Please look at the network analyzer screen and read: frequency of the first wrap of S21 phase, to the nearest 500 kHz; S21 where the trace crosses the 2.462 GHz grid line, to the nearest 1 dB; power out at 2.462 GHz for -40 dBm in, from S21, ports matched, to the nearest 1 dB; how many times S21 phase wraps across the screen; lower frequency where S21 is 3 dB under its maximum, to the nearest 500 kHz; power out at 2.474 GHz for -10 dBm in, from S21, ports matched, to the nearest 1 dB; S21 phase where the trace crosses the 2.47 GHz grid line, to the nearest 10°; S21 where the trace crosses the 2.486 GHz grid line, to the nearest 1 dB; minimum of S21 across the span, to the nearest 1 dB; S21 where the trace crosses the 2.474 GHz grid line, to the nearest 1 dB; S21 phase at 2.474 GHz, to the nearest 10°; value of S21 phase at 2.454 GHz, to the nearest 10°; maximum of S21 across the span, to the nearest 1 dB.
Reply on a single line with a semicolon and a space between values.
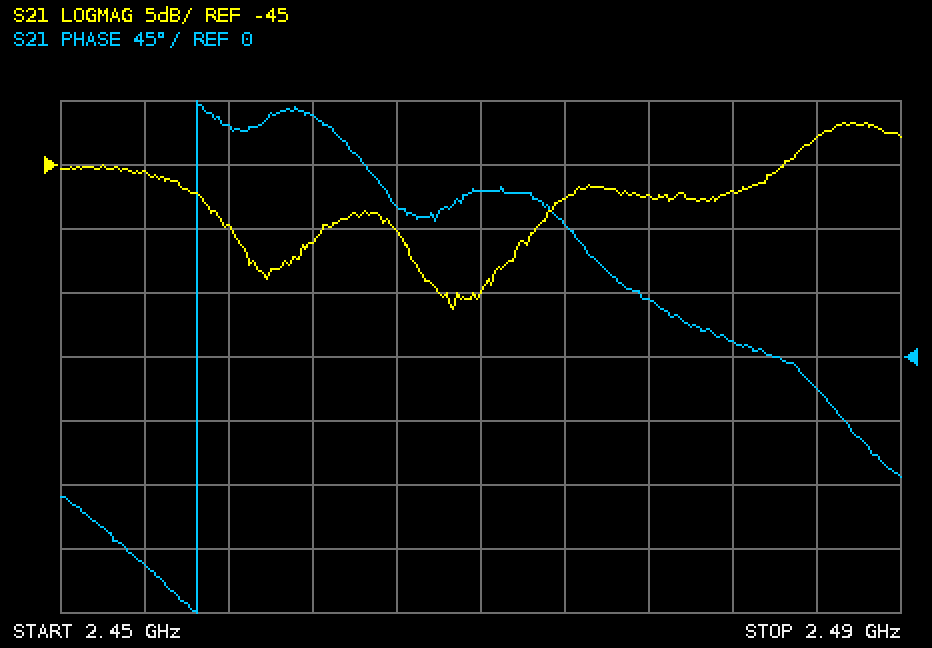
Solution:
2.4565 GHz; -51 dB; -91 dBm; 1; 2.4845 GHz; -58 dBm; 120°; -43 dB; -56 dB; -48 dB; 90°; -150°; -42 dB
